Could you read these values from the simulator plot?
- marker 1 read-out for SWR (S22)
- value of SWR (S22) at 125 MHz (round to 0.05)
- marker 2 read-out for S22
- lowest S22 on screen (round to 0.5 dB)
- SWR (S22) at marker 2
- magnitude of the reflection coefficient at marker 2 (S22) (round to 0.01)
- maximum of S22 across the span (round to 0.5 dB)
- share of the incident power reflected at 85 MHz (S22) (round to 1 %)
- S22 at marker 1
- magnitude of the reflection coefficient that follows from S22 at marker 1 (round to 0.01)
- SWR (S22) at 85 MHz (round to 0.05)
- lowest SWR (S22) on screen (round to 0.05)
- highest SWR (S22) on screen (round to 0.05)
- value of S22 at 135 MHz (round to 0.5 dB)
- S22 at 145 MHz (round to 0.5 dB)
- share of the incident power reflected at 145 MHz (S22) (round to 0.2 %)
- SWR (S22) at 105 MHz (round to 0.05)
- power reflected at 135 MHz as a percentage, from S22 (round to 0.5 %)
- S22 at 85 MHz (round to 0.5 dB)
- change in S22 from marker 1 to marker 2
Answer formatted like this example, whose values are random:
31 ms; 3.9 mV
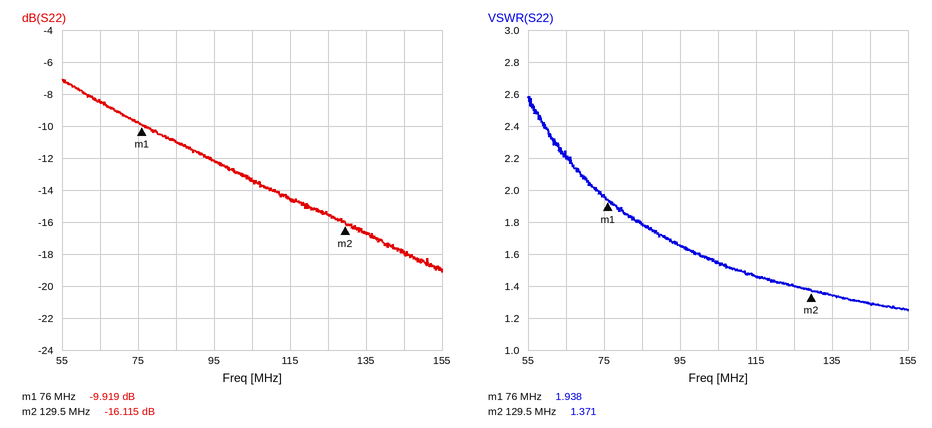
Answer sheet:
1.938; 1.40; -16.115 dB; -19.0 dB; 1.371; 0.16; -7.0 dB; 8 %; -9.919 dB; 0.32; 1.80; 1.25; 2.60; -16.5 dB; -18.0 dB; 1.6 %; 1.55; 2.0 %; -11.0 dB; -6.196 dB
